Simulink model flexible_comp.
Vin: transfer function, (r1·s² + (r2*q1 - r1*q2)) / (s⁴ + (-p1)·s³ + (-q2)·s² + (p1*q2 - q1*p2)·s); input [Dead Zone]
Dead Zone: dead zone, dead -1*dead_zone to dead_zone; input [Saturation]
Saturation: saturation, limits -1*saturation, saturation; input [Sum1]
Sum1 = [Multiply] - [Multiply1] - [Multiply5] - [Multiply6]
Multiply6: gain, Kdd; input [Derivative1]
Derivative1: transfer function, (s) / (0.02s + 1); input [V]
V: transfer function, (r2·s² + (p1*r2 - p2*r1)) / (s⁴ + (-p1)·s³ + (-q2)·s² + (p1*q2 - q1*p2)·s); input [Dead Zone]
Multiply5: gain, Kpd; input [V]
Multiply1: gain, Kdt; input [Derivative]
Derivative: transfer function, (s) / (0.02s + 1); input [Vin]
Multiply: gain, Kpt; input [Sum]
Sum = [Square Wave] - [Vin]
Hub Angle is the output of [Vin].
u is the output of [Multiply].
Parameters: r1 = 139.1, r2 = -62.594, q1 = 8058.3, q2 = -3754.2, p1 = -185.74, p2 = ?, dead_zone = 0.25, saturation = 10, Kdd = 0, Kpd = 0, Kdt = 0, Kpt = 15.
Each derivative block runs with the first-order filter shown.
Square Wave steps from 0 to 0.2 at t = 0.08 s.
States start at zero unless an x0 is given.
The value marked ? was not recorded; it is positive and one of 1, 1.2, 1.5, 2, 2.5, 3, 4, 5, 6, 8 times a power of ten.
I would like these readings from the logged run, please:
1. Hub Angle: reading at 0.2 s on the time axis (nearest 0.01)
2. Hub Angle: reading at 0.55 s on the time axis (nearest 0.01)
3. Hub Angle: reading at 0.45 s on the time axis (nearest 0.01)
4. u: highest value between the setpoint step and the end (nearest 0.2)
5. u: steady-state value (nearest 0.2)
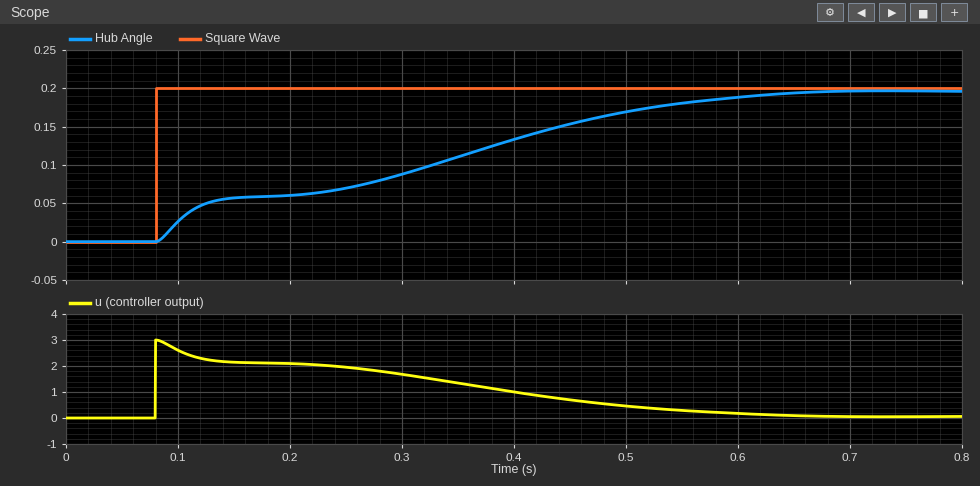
0.06
0.18
0.15
3.0
0.0
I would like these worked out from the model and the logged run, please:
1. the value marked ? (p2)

80
